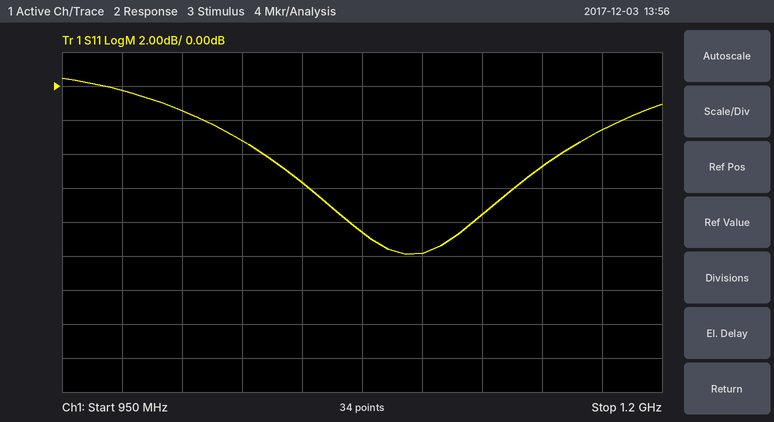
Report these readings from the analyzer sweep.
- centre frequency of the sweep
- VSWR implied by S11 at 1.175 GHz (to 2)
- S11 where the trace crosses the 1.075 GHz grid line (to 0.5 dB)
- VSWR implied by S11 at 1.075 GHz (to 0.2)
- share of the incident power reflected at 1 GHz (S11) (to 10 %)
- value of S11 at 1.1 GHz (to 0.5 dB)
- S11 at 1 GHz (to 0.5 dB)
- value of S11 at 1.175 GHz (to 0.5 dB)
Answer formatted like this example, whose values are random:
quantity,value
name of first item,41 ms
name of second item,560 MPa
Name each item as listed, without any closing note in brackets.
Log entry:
quantity,value
centre frequency of the sweep,1.075 GHz
VSWR implied by S11 at 1.175 GHz,6
S11 where the trace crosses the 1.075 GHz grid line,-8.5 dB
VSWR implied by S11 at 1.075 GHz,2.2
share of the incident power reflected at 1 GHz (S11),70 %
value of S11 at 1.1 GHz,-10.0 dB
S11 at 1 GHz,-1.5 dB
value of S11 at 1.175 GHz,-2.5 dB
